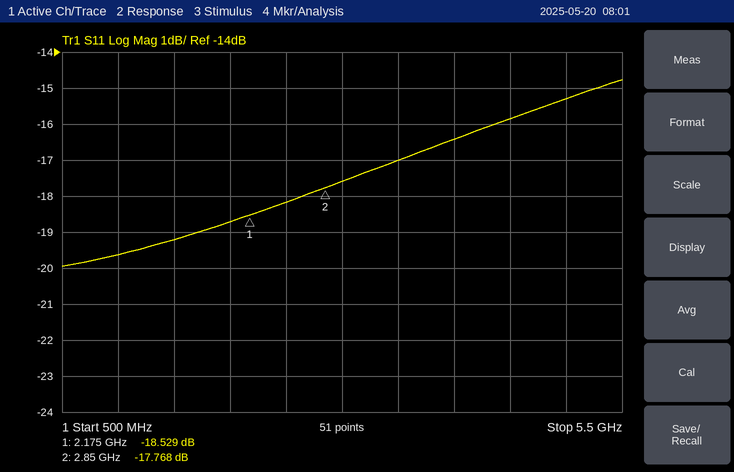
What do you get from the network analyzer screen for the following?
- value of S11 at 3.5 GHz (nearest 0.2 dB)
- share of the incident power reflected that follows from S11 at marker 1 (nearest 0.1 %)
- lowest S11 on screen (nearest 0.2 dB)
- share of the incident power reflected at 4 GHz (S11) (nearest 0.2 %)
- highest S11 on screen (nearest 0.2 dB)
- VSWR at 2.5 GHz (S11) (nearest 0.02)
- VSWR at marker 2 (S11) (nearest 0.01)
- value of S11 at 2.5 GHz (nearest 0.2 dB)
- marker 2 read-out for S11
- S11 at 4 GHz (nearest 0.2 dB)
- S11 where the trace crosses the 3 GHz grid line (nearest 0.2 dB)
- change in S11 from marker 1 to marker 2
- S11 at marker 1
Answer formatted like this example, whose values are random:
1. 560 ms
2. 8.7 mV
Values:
1. -17.0 dB
2. 1.4 %
3. -20.0 dB
4. 2.2 %
5. -14.8 dB
6. 1.28
7. 1.30
8. -18.2 dB
9. -17.768 dB
10. -16.4 dB
11. -17.6 dB
12. 0.761 dB
13. -18.529 dB
